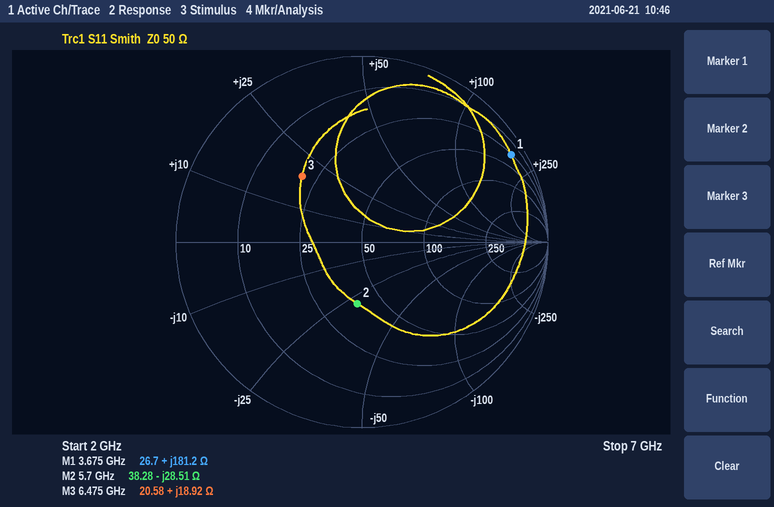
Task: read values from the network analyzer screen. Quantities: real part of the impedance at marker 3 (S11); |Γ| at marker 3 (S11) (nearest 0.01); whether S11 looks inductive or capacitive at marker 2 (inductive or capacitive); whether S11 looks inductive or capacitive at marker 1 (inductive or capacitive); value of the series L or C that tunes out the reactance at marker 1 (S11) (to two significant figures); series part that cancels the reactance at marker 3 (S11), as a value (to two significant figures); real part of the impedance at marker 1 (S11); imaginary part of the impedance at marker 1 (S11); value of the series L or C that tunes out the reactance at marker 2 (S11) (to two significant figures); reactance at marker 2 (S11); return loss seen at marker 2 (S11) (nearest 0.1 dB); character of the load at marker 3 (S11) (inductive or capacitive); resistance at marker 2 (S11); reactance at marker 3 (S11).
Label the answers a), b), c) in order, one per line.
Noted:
a) 20.58 Ω
b) 0.48
c) capacitive
d) inductive
e) 240 fF
f) 1.3 pF
g) 26.7 Ω
h) +181.2 Ω
i) 800 pH
j) -28.51 Ω
k) 9.6 dB
l) inductive
m) 38.28 Ω
n) +18.92 Ω
